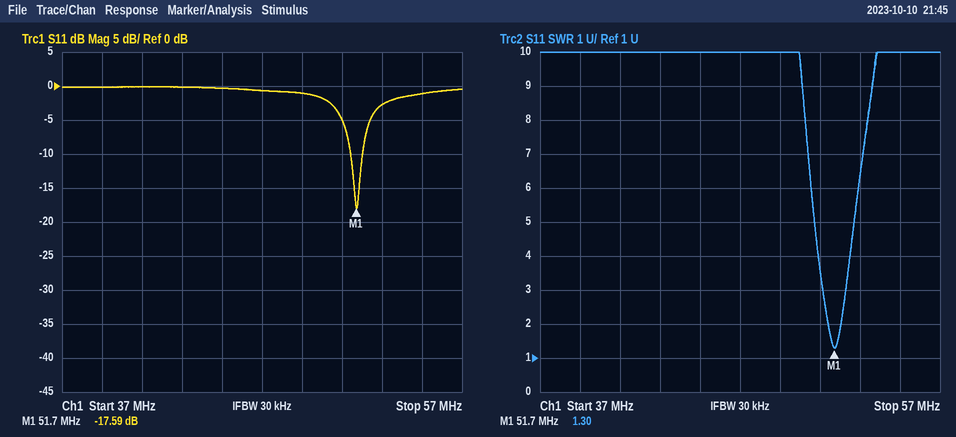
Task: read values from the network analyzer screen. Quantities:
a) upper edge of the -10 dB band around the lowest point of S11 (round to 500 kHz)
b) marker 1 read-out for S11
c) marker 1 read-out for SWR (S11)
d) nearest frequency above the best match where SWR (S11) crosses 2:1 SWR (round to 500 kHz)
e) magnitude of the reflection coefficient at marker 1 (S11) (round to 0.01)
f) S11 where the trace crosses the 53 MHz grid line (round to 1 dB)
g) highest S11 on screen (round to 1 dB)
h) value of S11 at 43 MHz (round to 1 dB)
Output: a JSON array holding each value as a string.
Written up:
["52.0 MHz", "-17.59 dB", "1.30", "52.0 MHz", "0.13", "-3 dB", "0 dB", "0 dB"]
